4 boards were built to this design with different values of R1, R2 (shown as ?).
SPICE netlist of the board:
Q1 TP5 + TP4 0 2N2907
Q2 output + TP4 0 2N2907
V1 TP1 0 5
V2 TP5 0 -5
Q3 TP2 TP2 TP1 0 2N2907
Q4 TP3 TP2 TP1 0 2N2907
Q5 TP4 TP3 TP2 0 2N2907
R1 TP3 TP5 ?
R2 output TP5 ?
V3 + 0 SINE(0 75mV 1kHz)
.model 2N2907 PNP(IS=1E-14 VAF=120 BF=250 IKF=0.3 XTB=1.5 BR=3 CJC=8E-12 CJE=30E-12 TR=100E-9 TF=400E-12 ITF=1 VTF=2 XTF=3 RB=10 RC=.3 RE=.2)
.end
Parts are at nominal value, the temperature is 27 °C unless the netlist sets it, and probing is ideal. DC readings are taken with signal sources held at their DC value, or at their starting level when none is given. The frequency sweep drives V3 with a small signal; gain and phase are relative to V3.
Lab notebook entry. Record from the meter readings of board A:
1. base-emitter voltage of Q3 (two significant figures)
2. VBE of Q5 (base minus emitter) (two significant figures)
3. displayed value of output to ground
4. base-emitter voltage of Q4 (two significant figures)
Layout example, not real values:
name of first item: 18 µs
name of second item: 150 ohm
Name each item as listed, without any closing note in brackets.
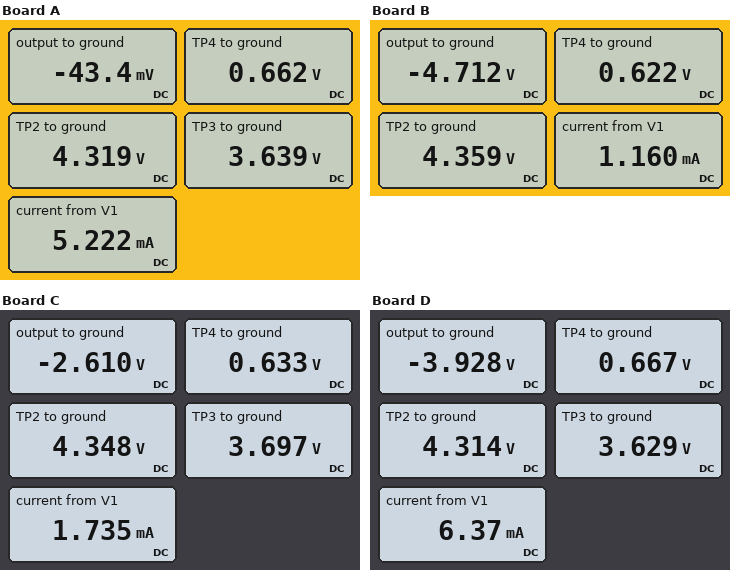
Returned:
base-emitter voltage of Q3: -680 mV
VBE of Q5 (base minus emitter): -680 mV
displayed value of output to ground: -43.4 mV
base-emitter voltage of Q4: -680 mV
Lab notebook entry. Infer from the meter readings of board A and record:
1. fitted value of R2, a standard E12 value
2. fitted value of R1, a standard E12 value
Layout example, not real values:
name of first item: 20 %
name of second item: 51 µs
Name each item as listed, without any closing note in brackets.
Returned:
fitted value of R2, a standard E12 value: 3.9 kΩ
fitted value of R1, a standard E12 value: 3.3 kΩ
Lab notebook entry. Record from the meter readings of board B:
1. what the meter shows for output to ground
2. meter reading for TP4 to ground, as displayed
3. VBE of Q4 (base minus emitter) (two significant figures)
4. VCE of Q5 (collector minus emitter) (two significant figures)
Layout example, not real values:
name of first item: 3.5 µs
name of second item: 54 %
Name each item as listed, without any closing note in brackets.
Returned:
what the meter shows for output to ground: -4.712 V
meter reading for TP4 to ground, as displayed: 0.622 V
VBE of Q4 (base minus emitter): -640 mV
VCE of Q5 (collector minus emitter): -3.7 V
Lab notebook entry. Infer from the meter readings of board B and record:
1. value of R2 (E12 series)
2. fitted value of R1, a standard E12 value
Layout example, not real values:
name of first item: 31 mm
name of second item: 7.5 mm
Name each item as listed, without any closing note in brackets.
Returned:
value of R2: 1 kΩ
fitted value of R1, a standard E12 value: 15 kΩ
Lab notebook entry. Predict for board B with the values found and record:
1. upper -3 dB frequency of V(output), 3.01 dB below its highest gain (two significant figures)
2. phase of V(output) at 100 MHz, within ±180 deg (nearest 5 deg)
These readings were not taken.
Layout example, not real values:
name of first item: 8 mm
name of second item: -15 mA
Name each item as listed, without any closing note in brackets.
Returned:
upper -3 dB frequency of V(output), 3.01 dB below its highest gain: 4.2 GHz
phase of V(output) at 100 MHz, within ±180 deg: 30 deg
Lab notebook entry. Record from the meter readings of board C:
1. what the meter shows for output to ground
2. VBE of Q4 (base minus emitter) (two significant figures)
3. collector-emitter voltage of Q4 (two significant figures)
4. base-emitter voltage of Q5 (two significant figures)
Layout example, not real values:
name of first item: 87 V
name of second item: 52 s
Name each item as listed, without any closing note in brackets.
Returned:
what the meter shows for output to ground: -2.610 V
VBE of Q4 (base minus emitter): -650 mV
collector-emitter voltage of Q4: -1.3 V
base-emitter voltage of Q5: -650 mV
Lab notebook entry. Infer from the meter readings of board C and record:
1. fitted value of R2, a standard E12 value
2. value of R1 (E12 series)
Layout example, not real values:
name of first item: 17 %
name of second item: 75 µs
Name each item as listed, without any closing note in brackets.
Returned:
fitted value of R2, a standard E12 value: 5.6 kΩ
value of R1: 10 kΩ
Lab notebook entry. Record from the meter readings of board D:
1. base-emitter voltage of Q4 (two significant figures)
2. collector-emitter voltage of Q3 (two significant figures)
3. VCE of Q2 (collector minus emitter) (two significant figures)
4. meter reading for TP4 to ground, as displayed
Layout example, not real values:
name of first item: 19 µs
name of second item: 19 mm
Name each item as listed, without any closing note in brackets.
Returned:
base-emitter voltage of Q4: -690 mV
collector-emitter voltage of Q3: -690 mV
VCE of Q2 (collector minus emitter): -4.6 V
meter reading for TP4 to ground, as displayed: 0.667 V
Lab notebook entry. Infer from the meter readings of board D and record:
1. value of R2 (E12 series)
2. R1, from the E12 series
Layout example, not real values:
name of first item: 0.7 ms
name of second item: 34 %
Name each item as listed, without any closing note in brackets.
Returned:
value of R2: 680 Ω
R1, from the E12 series: 2.7 kΩ
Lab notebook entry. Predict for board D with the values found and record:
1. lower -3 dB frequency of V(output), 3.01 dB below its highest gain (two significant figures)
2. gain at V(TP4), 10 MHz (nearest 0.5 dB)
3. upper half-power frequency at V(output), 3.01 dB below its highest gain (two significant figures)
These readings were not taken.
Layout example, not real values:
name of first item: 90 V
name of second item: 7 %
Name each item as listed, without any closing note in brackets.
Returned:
lower -3 dB frequency of V(output), 3.01 dB below its highest gain: 110 MHz
gain at V(TP4), 10 MHz: 0 dB
upper half-power frequency at V(output), 3.01 dB below its highest gain: 4.3 GHz
